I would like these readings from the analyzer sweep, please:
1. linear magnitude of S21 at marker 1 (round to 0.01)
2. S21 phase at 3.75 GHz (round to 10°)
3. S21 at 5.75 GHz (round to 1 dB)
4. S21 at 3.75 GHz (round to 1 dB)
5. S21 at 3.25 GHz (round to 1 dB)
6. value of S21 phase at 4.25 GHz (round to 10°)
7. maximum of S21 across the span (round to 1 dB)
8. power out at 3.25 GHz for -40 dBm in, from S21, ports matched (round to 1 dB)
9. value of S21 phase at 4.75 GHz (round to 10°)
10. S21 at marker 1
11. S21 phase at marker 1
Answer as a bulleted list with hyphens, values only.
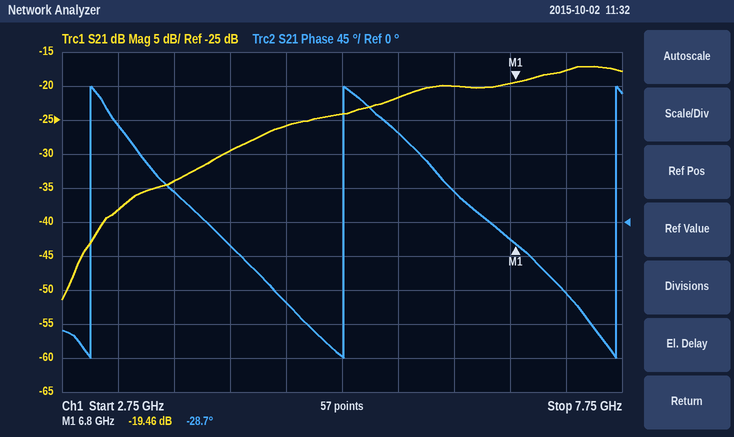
- 0.11
- 40°
- -22 dB
- -34 dB
- -38 dB
- -30°
- -17 dB
- -78 dBm
- -110°
- -19.46 dB
- -28.7°
